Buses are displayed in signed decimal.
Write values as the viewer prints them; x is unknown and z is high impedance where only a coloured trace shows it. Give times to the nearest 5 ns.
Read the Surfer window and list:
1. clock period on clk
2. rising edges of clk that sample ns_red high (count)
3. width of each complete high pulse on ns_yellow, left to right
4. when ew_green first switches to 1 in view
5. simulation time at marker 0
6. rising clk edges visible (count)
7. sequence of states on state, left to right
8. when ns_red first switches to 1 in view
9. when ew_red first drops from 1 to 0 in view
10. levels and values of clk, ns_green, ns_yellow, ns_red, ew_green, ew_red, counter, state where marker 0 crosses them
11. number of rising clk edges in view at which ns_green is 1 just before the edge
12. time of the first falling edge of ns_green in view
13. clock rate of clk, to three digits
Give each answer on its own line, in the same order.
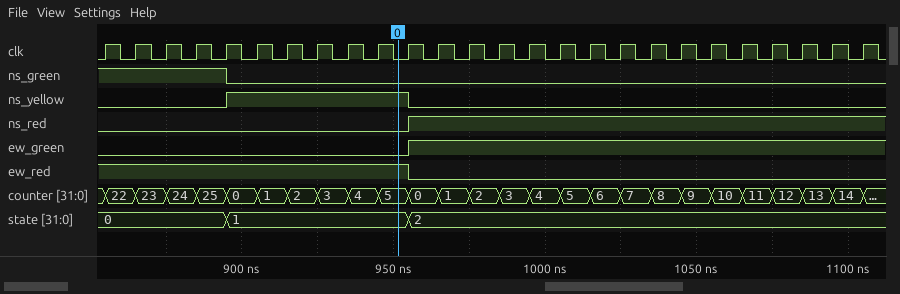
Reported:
10 ns
15
60 ns
955 ns
950 ns
26
0, 1, 2
955 ns
955 ns
clk=0, ns_green=0, ns_yellow=1, ns_red=0, ew_green=0, ew_red=1, counter=5, state=1
5
895 ns
100 MHz
